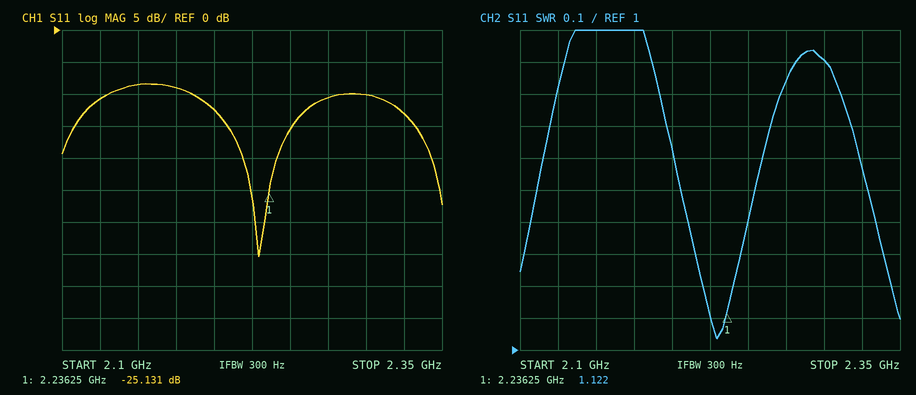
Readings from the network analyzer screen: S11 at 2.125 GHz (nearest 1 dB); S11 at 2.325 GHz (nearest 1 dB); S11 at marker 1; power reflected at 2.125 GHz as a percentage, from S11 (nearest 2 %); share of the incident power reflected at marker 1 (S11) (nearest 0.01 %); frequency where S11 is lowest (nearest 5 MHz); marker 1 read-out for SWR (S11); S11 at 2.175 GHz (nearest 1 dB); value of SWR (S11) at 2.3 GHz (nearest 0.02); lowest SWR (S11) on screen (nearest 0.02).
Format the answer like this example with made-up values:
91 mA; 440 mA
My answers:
-11 dB; -13 dB; -25.131 dB; 8 %; 0.31 %; 2.230 GHz; 1.122; -9 dB; 1.90; 1.04
